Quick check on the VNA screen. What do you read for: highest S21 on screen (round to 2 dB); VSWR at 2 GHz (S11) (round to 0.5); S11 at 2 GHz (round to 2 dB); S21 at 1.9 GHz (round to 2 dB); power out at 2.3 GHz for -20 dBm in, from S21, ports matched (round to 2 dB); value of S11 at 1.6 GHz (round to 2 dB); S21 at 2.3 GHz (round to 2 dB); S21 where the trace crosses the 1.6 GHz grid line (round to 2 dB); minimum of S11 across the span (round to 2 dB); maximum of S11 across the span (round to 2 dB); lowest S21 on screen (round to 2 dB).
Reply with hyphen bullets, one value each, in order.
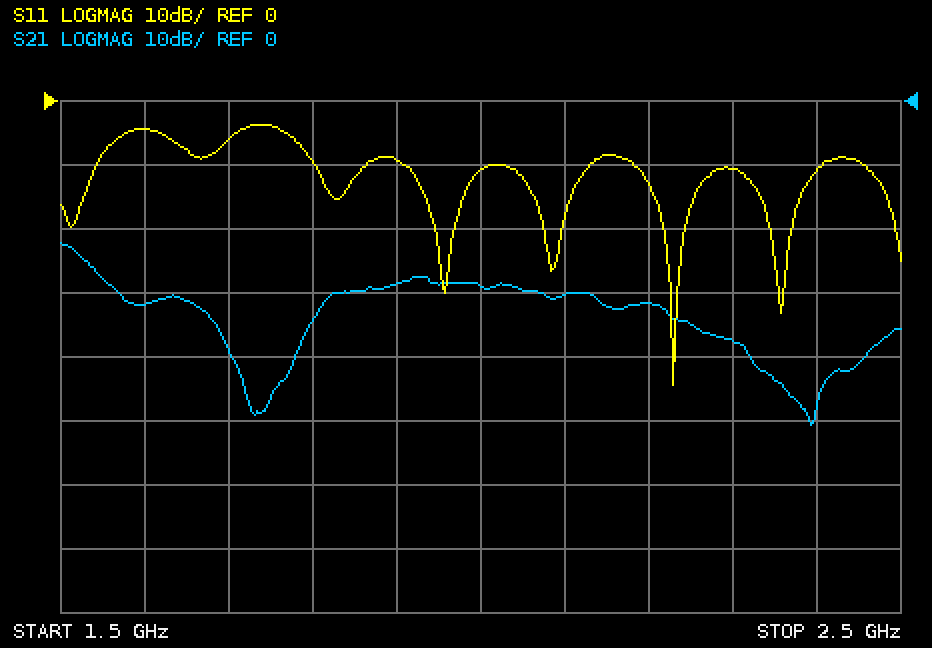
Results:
- -22 dB
- 2.0
- -10 dB
- -28 dB
- -58 dBm
- -4 dB
- -38 dB
- -32 dB
- -44 dB
- -4 dB
- -50 dB
